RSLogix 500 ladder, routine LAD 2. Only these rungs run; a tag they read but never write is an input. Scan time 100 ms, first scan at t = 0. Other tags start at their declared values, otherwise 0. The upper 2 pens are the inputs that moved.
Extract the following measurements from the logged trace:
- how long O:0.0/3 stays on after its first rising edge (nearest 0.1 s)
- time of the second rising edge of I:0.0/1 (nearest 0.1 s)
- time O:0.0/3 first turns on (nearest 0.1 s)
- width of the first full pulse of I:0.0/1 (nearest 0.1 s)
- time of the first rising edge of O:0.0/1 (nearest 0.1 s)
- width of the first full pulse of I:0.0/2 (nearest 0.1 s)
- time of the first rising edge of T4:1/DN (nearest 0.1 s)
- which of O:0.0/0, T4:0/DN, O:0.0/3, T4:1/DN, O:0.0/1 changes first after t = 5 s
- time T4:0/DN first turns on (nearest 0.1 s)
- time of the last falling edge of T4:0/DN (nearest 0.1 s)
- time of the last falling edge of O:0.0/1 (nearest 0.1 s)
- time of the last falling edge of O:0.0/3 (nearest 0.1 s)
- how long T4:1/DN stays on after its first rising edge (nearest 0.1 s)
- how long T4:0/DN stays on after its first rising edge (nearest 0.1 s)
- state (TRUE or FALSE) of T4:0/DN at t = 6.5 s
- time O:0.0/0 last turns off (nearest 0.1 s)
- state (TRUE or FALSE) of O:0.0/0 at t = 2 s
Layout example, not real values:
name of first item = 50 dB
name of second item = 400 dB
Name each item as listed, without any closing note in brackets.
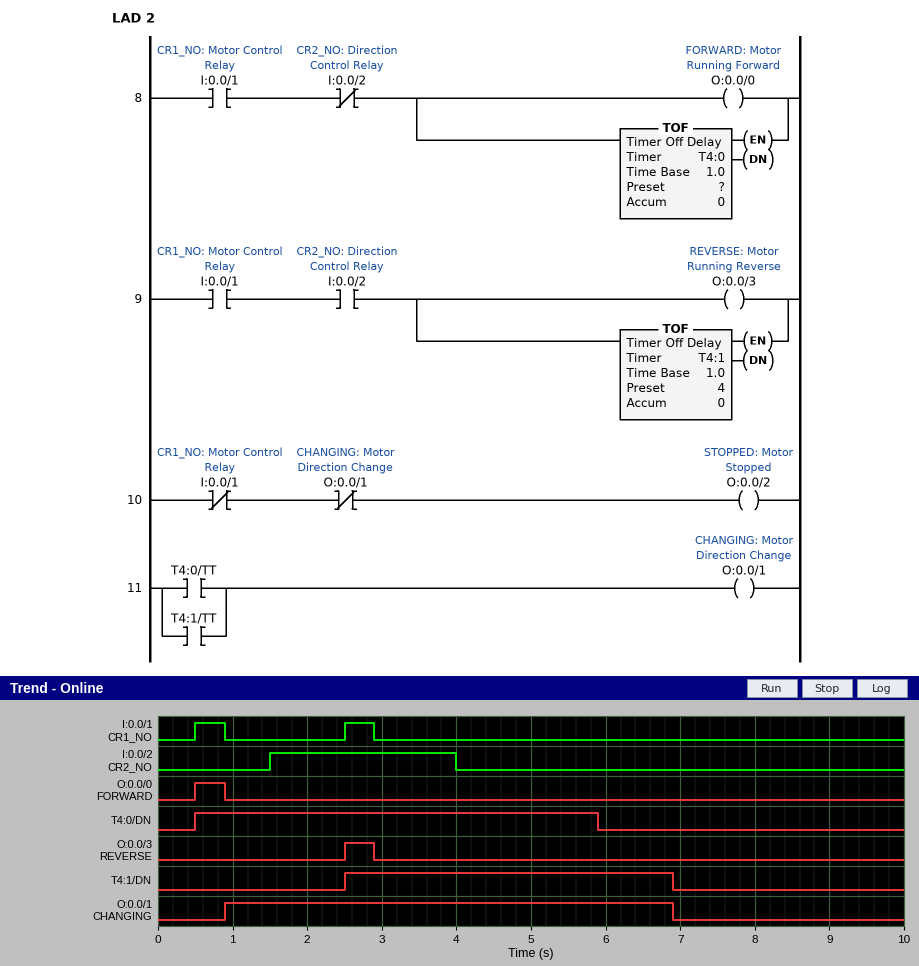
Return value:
how long O:0.0/3 stays on after its first rising edge = 0.4 s
time of the second rising edge of I:0.0/1 = 2.5 s
time O:0.0/3 first turns on = 2.5 s
width of the first full pulse of I:0.0/1 = 0.4 s
time of the first rising edge of O:0.0/1 = 0.9 s
width of the first full pulse of I:0.0/2 = 2.5 s
time of the first rising edge of T4:1/DN = 2.5 s
which of O:0.0/0, T4:0/DN, O:0.0/3, T4:1/DN, O:0.0/1 changes first after t = 5 s = T4:0/DN
time T4:0/DN first turns on = 0.5 s
time of the last falling edge of T4:0/DN = 5.9 s
time of the last falling edge of O:0.0/1 = 6.9 s
time of the last falling edge of O:0.0/3 = 2.9 s
how long T4:1/DN stays on after its first rising edge = 4.4 s
how long T4:0/DN stays on after its first rising edge = 5.4 s
state (TRUE or FALSE) of T4:0/DN at t = 6.5 s = FALSE
time O:0.0/0 last turns off = 0.9 s
state (TRUE or FALSE) of O:0.0/0 at t = 2 s = FALSE
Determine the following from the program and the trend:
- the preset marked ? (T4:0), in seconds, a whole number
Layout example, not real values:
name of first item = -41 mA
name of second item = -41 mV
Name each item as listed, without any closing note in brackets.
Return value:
the preset marked ? (T4:0), in seconds, a whole number = 5 s
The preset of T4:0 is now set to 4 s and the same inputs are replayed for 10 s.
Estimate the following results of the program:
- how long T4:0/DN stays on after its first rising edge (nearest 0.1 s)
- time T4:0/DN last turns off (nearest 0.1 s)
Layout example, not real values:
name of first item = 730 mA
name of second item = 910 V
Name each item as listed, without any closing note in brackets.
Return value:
how long T4:0/DN stays on after its first rising edge = 4.4 s
time T4:0/DN last turns off = 4.9 s
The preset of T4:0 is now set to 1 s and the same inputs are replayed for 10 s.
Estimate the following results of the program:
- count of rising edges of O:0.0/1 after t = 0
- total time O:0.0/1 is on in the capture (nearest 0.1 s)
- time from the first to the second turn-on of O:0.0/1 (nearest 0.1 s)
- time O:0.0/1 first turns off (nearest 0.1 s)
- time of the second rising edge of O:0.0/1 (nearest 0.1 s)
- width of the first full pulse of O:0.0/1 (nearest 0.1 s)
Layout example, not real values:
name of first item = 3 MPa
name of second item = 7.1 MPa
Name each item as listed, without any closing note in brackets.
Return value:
count of rising edges of O:0.0/1 after t = 0 = 2
total time O:0.0/1 is on in the capture = 5.0 s
time from the first to the second turn-on of O:0.0/1 = 2.0 s
time O:0.0/1 first turns off = 1.9 s
time of the second rising edge of O:0.0/1 = 2.9 s
width of the first full pulse of O:0.0/1 = 1.0 s
